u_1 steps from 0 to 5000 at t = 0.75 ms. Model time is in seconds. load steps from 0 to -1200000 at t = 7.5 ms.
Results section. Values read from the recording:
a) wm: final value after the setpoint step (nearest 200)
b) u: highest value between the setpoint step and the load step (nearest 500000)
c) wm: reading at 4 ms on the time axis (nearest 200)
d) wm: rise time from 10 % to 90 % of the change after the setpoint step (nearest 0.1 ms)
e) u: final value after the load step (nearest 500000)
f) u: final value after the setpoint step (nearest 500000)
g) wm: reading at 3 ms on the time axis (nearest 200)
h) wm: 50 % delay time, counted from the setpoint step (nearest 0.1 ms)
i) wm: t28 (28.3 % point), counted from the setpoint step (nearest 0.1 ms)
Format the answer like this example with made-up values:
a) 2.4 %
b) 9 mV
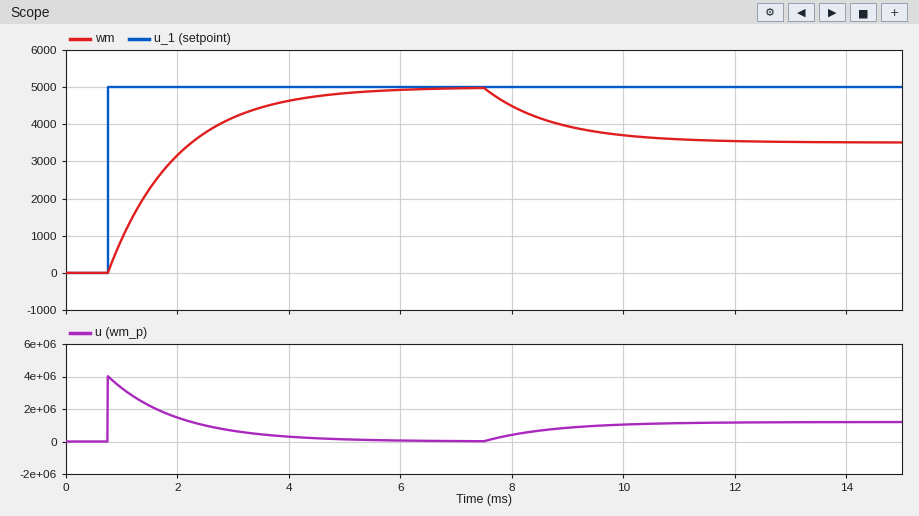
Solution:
a) 5000
b) 4000000
c) 4600
d) 2.7 ms
e) 1000000
f) 0
g) 4200
h) 0.9 ms
i) 0.4 ms
